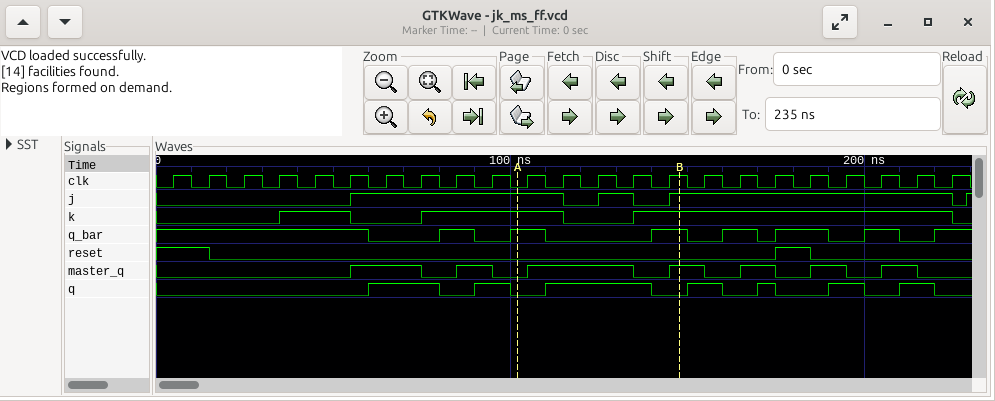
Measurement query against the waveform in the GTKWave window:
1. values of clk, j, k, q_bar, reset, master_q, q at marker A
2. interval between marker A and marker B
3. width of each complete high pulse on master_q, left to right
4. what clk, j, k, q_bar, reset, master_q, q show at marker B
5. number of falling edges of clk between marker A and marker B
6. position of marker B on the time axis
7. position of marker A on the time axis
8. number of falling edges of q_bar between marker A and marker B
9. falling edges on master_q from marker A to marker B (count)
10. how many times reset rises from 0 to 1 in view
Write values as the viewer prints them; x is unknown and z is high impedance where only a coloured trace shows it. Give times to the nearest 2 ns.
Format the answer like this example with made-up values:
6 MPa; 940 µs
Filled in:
clk=0, j=1, k=1, q_bar=1, reset=0, master_q=0, q=0; 46 ns; 20 ns, 10 ns, 30 ns, 10 ns, 10 ns, 10 ns, 10 ns; clk=1, j=1, k=1, q_bar=1, reset=0, master_q=1, q=0; 4; 148 ns; 102 ns; 1; 1; 1
